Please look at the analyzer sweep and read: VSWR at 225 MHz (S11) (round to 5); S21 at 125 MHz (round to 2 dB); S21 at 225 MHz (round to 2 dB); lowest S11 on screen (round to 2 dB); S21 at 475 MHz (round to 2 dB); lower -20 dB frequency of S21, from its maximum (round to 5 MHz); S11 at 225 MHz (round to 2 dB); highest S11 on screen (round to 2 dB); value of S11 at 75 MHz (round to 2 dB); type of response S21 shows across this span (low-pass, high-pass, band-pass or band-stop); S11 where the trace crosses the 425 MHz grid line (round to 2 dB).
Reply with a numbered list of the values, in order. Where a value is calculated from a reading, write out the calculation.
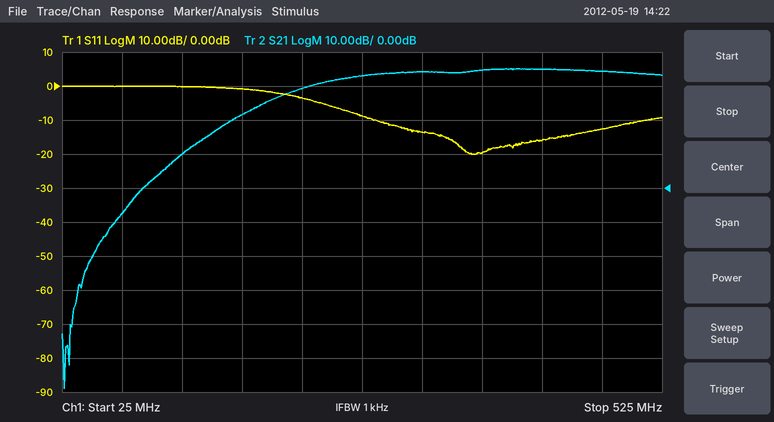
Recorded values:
1. |Γ| = 10^(-4/20) = 0.6310; VSWR = (1 + 0.6310)/(1 − 0.6310) ≈ 4.42, so 5 to the nearest 5
2. 10 dB
3. 30 dB
4. -20 dB
5. 34 dB
6. 145 MHz
7. -4 dB
8. 0 dB
9. 0 dB
10. high-pass
11. -16 dB
